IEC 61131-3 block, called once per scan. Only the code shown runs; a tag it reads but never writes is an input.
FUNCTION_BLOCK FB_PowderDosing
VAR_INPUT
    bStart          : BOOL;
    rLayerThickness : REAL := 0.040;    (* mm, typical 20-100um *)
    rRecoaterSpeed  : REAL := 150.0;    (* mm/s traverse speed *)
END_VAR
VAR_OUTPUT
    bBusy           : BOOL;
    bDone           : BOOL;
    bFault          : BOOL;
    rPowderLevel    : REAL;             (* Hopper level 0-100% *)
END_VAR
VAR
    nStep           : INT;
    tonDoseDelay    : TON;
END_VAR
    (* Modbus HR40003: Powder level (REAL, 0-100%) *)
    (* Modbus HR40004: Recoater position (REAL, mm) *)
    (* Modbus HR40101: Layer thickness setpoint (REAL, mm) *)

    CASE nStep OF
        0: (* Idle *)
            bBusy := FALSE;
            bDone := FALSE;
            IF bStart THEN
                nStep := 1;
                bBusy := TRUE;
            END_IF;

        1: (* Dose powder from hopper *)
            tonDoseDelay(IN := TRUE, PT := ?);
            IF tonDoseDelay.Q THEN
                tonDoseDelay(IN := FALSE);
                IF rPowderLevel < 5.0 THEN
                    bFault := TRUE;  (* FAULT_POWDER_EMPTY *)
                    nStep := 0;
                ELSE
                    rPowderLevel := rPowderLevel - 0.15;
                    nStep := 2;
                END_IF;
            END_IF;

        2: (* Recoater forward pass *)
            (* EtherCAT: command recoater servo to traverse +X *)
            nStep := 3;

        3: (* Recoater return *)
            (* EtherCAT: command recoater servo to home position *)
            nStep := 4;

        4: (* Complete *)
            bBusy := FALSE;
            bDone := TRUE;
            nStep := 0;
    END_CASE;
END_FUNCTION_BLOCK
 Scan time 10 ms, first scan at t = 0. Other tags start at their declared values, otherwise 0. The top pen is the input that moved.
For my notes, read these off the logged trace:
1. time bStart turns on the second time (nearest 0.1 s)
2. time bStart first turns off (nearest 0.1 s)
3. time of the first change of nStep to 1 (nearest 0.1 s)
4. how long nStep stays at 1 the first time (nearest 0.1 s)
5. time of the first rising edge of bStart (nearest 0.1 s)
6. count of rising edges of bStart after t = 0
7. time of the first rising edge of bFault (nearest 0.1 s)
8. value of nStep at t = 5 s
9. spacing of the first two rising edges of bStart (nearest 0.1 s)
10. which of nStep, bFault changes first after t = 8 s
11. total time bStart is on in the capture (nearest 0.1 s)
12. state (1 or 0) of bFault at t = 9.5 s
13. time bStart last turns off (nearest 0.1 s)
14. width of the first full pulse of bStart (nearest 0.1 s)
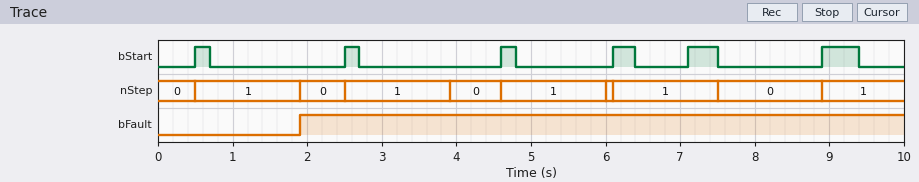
2.5 s
0.7 s
0.5 s
1.4 s
0.5 s
6
1.9 s
1
2.0 s
nStep
1.8 s
1
9.4 s
0.2 s
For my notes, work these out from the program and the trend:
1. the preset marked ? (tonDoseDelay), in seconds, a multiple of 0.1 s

1.4 s
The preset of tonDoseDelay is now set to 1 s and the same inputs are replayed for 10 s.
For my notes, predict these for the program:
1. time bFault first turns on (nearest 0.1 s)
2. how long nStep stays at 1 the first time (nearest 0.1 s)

1.5 s
1.0 s
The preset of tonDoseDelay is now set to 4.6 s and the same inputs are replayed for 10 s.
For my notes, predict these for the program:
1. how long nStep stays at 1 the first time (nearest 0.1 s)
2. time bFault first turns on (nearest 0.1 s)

4.6 s
5.1 s
